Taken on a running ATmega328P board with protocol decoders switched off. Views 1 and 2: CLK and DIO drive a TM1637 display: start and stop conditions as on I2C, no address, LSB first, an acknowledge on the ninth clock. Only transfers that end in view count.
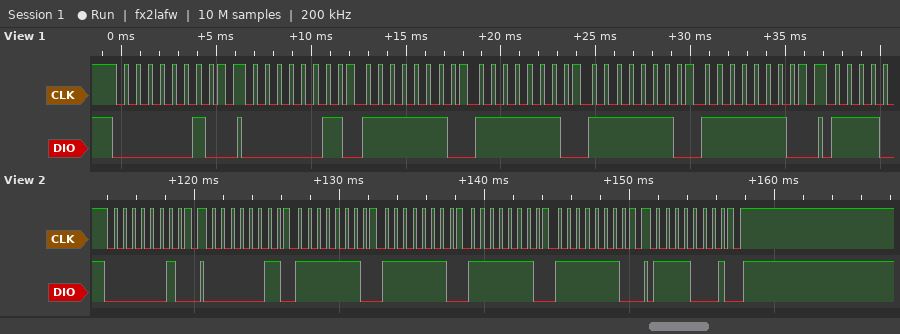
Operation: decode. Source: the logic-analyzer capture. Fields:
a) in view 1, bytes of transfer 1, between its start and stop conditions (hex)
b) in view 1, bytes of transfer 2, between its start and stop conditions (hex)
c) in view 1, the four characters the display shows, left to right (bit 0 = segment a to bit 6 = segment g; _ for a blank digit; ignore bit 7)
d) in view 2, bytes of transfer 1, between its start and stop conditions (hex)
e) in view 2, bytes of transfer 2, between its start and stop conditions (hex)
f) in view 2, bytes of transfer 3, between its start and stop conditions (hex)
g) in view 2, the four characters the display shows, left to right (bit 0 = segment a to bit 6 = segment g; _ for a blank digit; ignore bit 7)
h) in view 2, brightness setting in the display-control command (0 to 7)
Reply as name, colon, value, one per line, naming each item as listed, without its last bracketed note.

in view 1, bytes of transfer 1, between its start and stop conditions: 40
in view 1, bytes of transfer 2, between its start and stop conditions: C0 7F 7F 7F 7F
in view 1, the four characters the display shows, left to right: 8888
in view 2, bytes of transfer 1, between its start and stop conditions: 40
in view 2, bytes of transfer 2, between its start and stop conditions: C0 7F 7F 7F 7F
in view 2, bytes of transfer 3, between its start and stop conditions: 8F
in view 2, the four characters the display shows, left to right: 8888
in view 2, brightness setting in the display-control command: 7
